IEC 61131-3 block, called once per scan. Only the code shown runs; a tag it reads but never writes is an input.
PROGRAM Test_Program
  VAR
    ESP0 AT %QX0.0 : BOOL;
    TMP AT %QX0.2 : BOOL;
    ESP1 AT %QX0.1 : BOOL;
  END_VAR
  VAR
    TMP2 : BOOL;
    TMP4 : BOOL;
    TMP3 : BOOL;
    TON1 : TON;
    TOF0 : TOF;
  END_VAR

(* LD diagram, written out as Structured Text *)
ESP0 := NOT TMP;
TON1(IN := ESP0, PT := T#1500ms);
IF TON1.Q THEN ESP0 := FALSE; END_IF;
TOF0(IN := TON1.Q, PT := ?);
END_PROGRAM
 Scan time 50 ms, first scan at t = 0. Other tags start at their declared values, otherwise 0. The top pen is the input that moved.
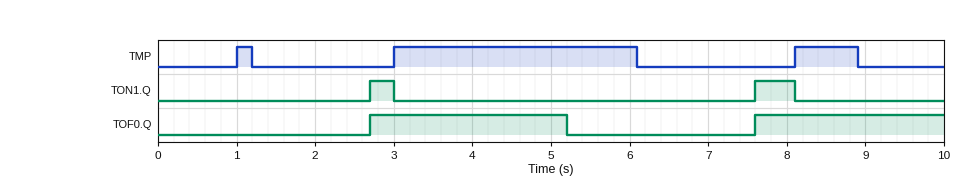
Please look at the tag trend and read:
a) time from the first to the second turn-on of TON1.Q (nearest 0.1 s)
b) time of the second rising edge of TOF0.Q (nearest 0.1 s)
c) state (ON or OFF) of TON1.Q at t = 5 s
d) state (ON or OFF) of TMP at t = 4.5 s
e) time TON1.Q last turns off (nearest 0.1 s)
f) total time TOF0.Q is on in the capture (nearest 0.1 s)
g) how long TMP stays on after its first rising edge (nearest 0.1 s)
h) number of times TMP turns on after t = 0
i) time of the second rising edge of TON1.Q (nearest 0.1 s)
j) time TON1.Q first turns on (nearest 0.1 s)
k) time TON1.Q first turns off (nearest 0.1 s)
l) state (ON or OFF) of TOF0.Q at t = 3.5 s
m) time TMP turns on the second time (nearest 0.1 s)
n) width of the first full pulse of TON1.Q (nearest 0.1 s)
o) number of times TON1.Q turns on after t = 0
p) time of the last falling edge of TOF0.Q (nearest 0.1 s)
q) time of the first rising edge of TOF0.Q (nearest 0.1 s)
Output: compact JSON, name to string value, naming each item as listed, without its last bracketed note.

{"time from the first to the second turn-on of TON1.Q": "4.9 s", "time of the second rising edge of TOF0.Q": "7.6 s", "state (ON or OFF) of TON1.Q at t = 5 s": "OFF", "state (ON or OFF) of TMP at t = 4.5 s": "ON", "time TON1.Q last turns off": "8.1 s", "total time TOF0.Q is on in the capture": "4.9 s", "how long TMP stays on after its first rising edge": "0.2 s", "number of times TMP turns on after t = 0": "3", "time of the second rising edge of TON1.Q": "7.6 s", "time TON1.Q first turns on": "2.7 s", "time TON1.Q first turns off": "3.0 s", "state (ON or OFF) of TOF0.Q at t = 3.5 s": "ON", "time TMP turns on the second time": "3.0 s", "width of the first full pulse of TON1.Q": "0.3 s", "number of times TON1.Q turns on after t = 0": "2", "time of the last falling edge of TOF0.Q": "5.2 s", "time of the first rising edge of TOF0.Q": "2.7 s"}
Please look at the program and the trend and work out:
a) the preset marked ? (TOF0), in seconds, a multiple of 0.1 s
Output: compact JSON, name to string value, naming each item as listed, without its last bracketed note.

{"the preset marked ? (TOF0), in seconds, a multiple of 0.1 s": "2.2 s"}
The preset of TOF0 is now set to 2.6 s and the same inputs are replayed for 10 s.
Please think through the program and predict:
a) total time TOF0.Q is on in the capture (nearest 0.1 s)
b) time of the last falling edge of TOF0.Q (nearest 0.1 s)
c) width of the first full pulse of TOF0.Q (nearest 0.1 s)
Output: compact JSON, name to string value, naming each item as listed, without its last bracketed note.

{"total time TOF0.Q is on in the capture": "5.3 s", "time of the last falling edge of TOF0.Q": "5.6 s", "width of the first full pulse of TOF0.Q": "2.9 s"}
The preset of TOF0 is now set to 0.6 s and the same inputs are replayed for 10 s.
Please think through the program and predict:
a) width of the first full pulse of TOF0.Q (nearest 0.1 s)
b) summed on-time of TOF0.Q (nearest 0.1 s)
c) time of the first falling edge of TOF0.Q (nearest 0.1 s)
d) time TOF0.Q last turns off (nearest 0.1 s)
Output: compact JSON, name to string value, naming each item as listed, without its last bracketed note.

{"width of the first full pulse of TOF0.Q": "0.9 s", "summed on-time of TOF0.Q": "2.0 s", "time of the first falling edge of TOF0.Q": "3.6 s", "time TOF0.Q last turns off": "8.7 s"}
